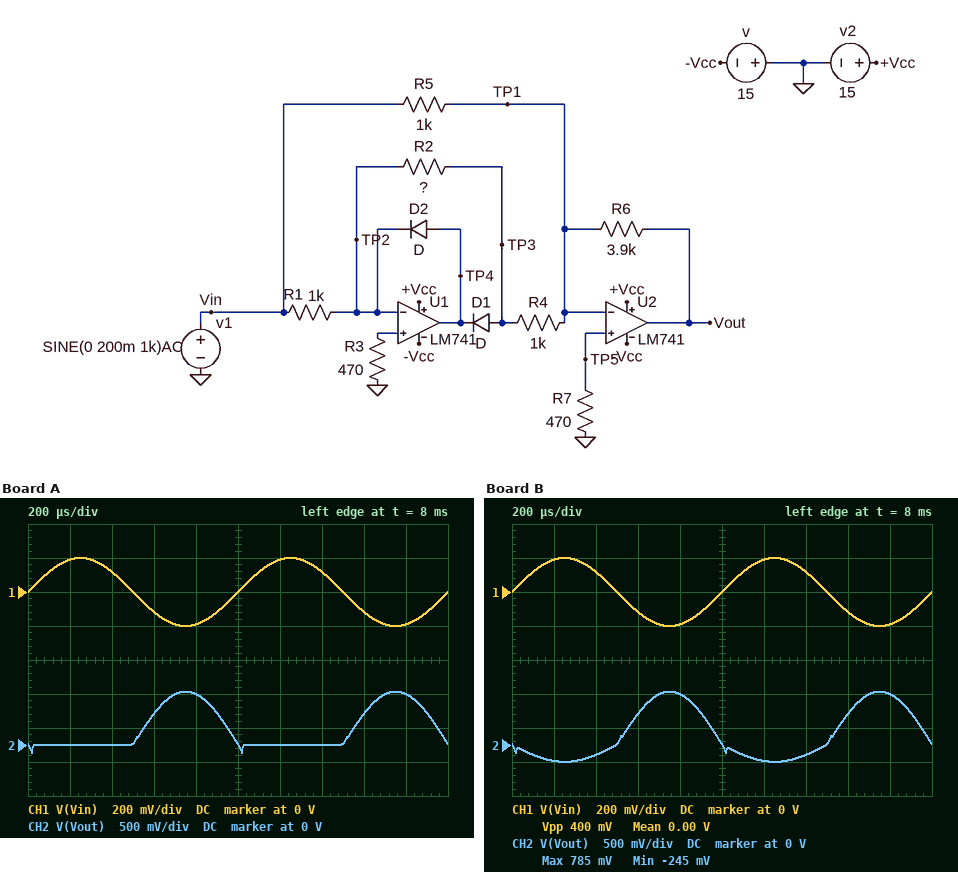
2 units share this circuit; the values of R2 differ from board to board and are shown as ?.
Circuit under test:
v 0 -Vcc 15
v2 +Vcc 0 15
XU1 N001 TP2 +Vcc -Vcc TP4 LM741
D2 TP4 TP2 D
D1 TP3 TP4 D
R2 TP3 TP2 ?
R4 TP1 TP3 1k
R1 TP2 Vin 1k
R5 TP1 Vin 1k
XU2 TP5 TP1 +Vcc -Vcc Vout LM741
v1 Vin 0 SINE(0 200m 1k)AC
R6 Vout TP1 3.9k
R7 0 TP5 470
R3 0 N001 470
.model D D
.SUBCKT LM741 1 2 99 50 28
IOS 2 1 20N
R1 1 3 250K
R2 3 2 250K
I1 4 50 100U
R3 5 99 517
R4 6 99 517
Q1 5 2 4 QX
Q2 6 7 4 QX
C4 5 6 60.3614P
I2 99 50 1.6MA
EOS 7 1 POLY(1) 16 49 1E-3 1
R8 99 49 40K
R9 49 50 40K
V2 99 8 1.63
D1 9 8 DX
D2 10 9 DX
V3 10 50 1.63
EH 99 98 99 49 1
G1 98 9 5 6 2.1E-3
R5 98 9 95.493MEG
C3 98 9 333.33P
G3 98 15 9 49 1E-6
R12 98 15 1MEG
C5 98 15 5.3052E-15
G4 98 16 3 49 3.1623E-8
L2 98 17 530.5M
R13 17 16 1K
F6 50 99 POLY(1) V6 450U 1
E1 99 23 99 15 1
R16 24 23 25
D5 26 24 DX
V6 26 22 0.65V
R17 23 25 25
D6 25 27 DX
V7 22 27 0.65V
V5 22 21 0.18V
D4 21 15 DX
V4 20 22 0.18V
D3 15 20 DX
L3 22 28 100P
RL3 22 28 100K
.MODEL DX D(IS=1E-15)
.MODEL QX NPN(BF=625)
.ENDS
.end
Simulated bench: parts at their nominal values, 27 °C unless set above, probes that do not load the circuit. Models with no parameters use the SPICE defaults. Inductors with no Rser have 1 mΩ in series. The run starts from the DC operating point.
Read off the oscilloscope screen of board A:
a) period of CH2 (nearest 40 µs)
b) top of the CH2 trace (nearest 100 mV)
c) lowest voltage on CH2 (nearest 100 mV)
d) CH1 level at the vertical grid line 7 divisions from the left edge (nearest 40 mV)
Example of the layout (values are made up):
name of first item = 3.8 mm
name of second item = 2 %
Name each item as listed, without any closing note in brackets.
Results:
period of CH2 = 1.00 ms
top of the CH2 trace = 800 mV
lowest voltage on CH2 = -100 mV
CH1 level at the vertical grid line 7 divisions from the left edge = 120 mV
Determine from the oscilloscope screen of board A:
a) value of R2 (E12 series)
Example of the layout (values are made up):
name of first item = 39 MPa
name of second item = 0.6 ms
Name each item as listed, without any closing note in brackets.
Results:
value of R2 = 1 kΩ
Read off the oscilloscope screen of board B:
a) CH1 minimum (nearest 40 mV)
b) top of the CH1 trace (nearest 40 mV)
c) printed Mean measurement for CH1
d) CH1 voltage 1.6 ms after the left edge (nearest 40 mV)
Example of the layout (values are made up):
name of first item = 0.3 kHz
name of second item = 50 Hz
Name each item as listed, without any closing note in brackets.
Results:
CH1 minimum = -200 mV
top of the CH1 trace = 200 mV
printed Mean measurement for CH1 = 0.00 V
CH1 voltage 1.6 ms after the left edge = -120 mV
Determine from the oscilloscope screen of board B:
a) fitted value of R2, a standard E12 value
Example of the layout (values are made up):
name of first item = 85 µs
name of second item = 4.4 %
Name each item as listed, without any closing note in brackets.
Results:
fitted value of R2, a standard E12 value = 680 Ω
